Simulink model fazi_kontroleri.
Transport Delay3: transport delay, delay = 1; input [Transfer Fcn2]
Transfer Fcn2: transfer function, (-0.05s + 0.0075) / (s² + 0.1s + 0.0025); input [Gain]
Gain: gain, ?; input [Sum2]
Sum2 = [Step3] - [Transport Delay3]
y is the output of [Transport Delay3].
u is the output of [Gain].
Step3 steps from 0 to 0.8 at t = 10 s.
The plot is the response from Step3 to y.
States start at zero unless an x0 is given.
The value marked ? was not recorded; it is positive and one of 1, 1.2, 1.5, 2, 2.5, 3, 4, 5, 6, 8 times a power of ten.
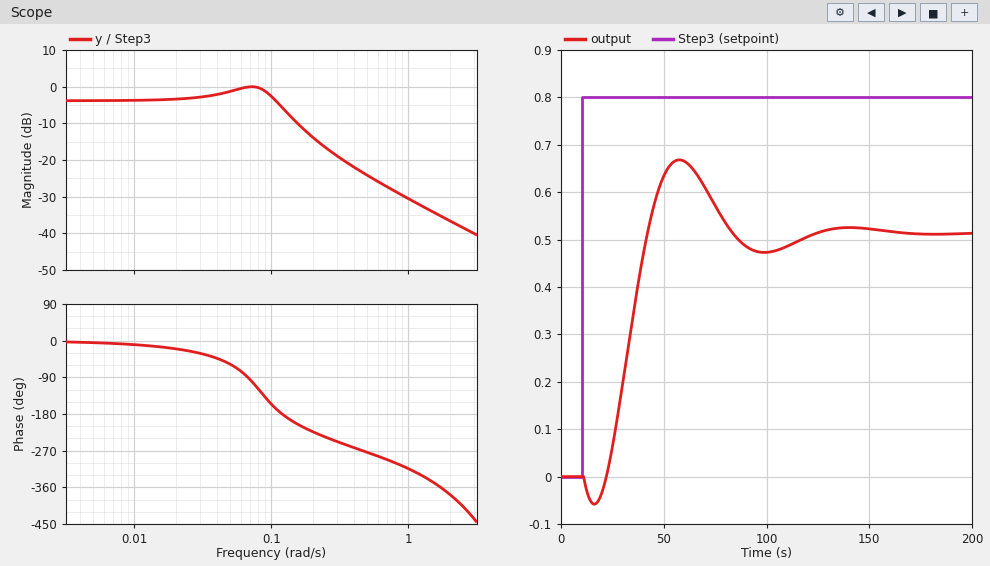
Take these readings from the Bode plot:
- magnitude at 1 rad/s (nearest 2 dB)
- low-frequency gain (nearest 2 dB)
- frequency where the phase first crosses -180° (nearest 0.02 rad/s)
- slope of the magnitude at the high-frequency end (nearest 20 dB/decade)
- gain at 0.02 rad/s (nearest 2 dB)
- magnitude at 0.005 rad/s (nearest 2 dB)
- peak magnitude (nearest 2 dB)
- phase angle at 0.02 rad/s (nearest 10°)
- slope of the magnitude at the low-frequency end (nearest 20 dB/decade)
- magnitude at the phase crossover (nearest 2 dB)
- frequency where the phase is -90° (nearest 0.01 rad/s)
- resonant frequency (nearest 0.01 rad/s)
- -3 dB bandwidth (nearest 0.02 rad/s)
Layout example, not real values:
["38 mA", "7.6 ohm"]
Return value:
["-30 dB", "-4 dB", "0.12 rad/s", "-20 dB/decade", "-4 dB", "-4 dB", "0 dB", "-20°", "0 dB/decade", "-6 dB", "0.07 rad/s", "0.07 rad/s", "0.12 rad/s"]
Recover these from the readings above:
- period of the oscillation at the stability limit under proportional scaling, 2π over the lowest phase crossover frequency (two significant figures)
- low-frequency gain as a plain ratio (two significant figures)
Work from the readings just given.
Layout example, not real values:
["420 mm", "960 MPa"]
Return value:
["52 s", "0.63"]
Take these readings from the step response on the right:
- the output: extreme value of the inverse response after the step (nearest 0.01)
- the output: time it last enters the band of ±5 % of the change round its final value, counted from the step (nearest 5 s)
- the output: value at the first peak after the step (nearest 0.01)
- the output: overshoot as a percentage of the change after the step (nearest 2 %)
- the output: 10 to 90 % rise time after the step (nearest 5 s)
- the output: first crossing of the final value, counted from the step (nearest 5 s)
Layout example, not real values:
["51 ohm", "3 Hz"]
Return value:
["-0.06", "100 s", "0.67", "30 %", "15 s", "30 s"]
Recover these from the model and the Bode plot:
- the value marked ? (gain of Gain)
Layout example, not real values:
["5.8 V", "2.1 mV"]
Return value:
["0.6"]
